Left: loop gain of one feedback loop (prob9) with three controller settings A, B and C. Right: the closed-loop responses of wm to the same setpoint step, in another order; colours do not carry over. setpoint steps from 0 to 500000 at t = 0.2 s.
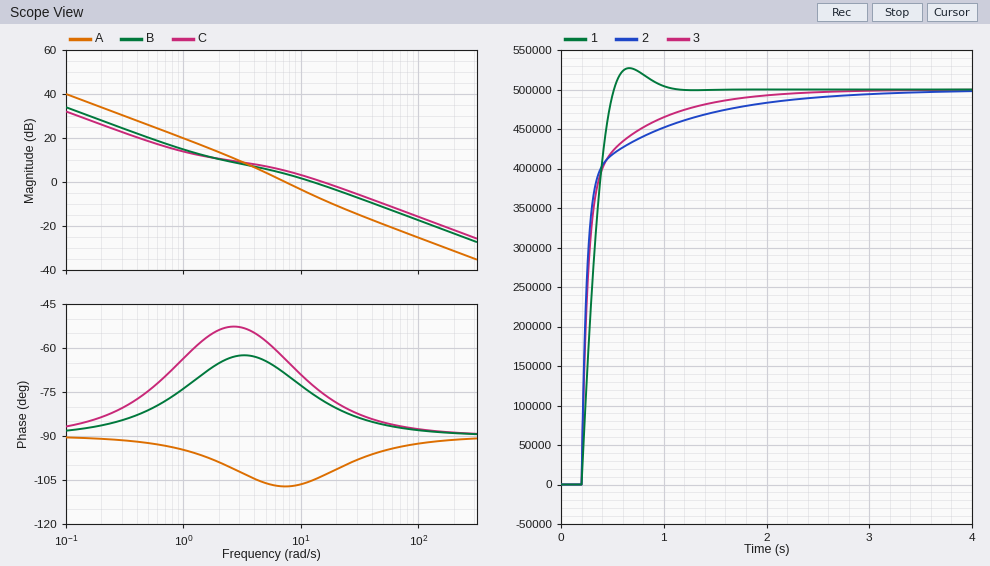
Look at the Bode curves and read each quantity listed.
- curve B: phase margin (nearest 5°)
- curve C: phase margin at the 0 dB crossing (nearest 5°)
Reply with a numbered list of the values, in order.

1. 105°
2. 105°
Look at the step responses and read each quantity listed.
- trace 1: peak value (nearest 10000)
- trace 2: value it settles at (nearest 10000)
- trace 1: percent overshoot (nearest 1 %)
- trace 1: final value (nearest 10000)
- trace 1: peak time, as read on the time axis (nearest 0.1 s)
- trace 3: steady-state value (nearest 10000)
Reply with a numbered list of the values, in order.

1. 530000
2. 500000
3. 5 %
4. 500000
5. 0.7 s
6. 500000
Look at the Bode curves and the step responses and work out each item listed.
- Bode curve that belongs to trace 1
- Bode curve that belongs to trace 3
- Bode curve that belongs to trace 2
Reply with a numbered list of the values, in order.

1. A
2. B
3. C
